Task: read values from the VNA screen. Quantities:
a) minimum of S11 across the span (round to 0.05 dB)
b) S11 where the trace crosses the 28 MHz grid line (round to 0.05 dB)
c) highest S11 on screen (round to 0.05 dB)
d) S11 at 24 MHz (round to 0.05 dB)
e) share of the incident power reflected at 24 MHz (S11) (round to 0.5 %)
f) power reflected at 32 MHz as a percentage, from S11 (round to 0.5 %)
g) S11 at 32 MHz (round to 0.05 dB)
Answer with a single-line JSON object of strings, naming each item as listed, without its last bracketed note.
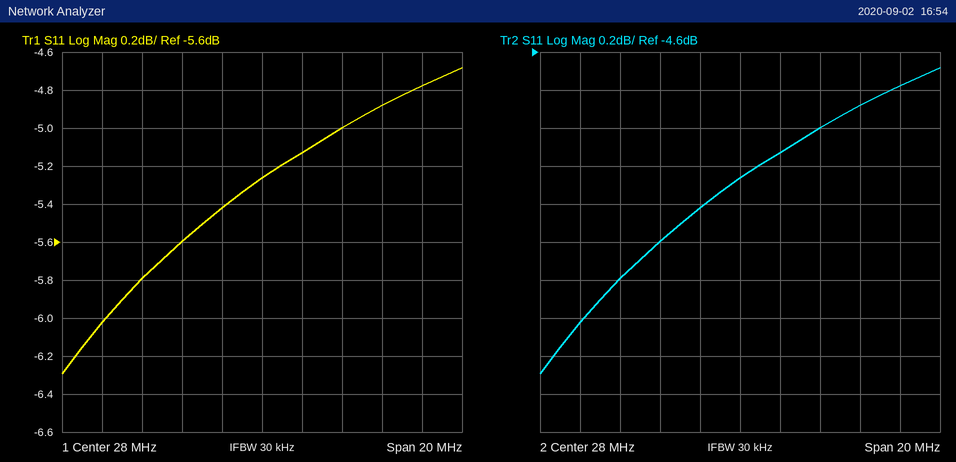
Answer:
{"minimum of S11 across the span": "-6.30 dB", "S11 where the trace crosses the 28 MHz grid line": "-5.25 dB", "highest S11 on screen": "-4.70 dB", "S11 at 24 MHz": "-5.60 dB", "share of the incident power reflected at 24 MHz (S11)": "27.5 %", "power reflected at 32 MHz as a percentage, from S11": "31.5 %", "S11 at 32 MHz": "-5.00 dB"}
